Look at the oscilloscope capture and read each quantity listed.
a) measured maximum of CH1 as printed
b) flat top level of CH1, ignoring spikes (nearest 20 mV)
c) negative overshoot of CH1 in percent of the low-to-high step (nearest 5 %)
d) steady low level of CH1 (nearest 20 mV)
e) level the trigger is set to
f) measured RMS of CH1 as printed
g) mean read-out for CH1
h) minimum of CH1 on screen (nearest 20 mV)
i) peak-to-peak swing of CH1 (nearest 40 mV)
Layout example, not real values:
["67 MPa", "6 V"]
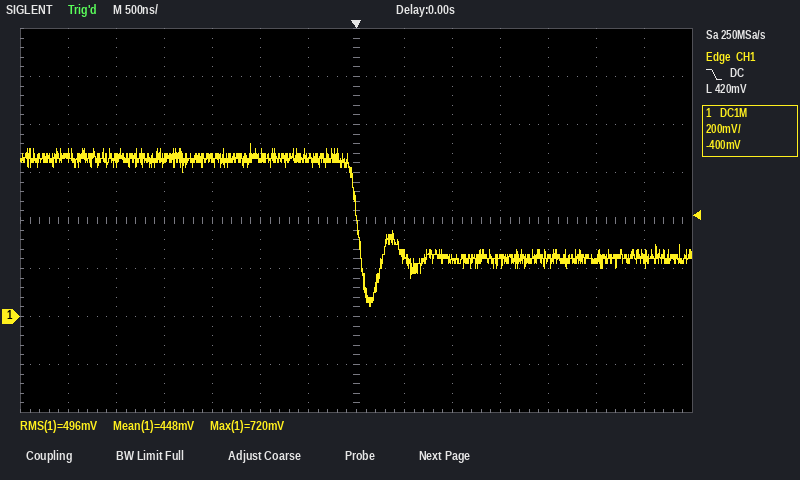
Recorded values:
["720 mV", "660 mV", "50 %", "240 mV", "420 mV", "496 mV", "448 mV", "40 mV", "680 mV"]
